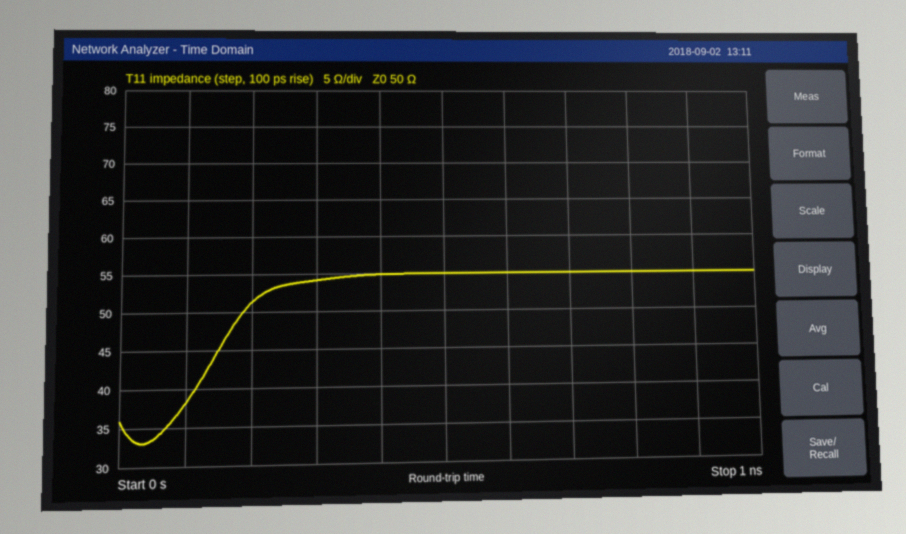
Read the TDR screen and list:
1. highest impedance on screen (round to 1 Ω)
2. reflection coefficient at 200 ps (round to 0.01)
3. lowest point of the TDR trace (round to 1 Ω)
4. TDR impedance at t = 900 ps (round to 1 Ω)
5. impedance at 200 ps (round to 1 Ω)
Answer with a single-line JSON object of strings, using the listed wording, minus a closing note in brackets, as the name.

{"highest impedance on screen": "55 Ω", "reflection coefficient at 200 ps": "+0.01", "lowest point of the TDR trace": "33 Ω", "TDR impedance at t = 900 ps": "55 Ω", "impedance at 200 ps": "51 Ω"}
